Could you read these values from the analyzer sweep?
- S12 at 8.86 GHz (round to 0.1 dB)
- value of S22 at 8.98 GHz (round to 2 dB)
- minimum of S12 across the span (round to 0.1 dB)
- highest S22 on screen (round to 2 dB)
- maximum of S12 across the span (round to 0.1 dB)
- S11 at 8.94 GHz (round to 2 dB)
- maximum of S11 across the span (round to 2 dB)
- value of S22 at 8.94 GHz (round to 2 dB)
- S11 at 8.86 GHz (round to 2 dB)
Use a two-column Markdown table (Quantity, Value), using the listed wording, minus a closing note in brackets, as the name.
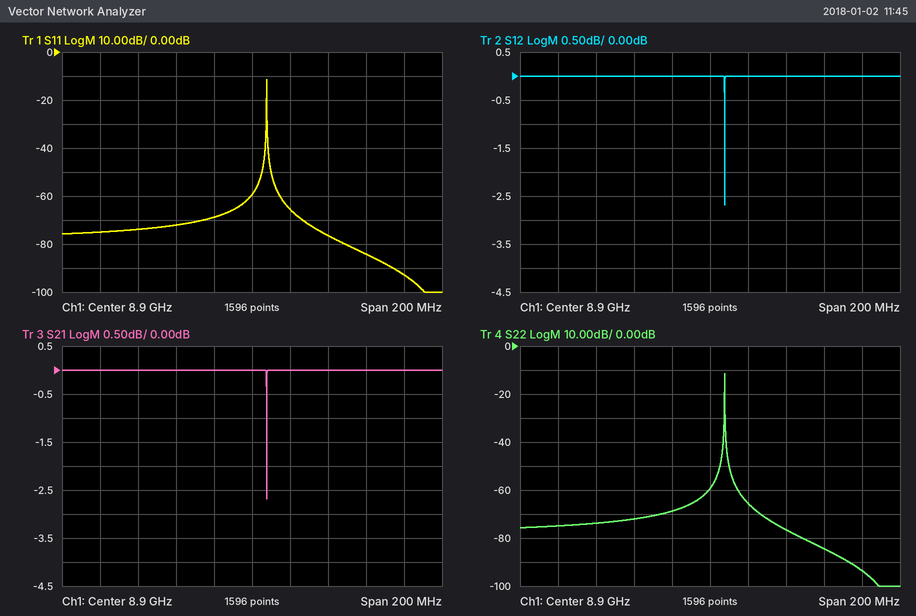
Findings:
| Quantity | Value |
|---|---|
| S12 at 8.86 GHz | 0.0 dB |
| value of S22 at 8.98 GHz | -94 dB |
| minimum of S12 across the span | -2.7 dB |
| highest S22 on screen | -12 dB |
| maximum of S12 across the span | 0.0 dB |
| S11 at 8.94 GHz | -76 dB |
| maximum of S11 across the span | -12 dB |
| value of S22 at 8.94 GHz | -76 dB |
| S11 at 8.86 GHz | -72 dB |
